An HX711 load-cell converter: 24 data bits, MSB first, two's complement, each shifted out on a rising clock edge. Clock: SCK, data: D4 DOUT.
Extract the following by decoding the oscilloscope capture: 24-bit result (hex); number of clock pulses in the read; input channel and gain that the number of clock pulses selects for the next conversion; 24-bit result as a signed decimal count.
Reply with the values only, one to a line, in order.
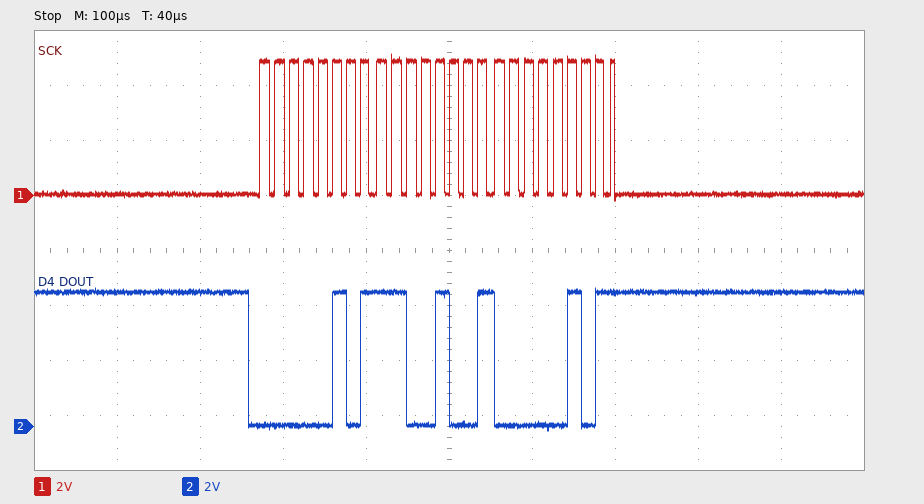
0x05C905
25
channel A, gain 128
379141
